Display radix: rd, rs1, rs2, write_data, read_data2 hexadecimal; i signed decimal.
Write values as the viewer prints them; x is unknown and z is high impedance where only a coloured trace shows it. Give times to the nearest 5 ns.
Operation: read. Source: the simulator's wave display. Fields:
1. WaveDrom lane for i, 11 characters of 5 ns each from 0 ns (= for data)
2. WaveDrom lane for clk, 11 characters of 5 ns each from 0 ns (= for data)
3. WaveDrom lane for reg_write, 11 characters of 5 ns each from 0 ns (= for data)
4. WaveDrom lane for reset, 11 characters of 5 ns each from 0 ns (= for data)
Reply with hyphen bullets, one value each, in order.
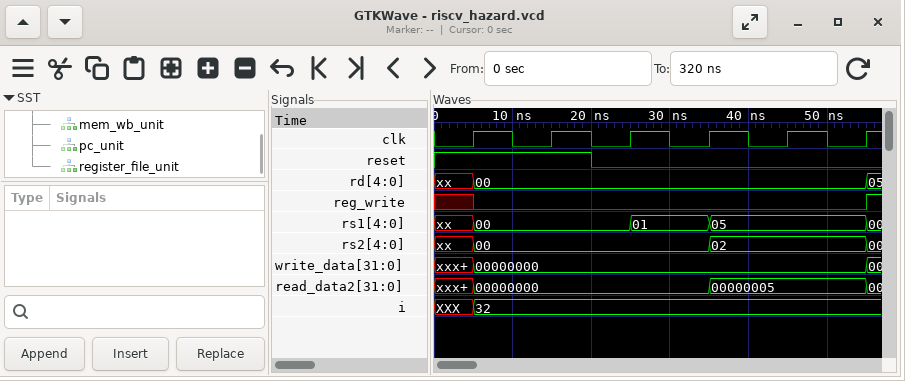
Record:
- {name: 'i', wave: 'x=.........', data: '32'}
- {name: 'clk', wave: '01010101010'}
- {name: 'reg_write', wave: 'x0.........'}
- {name: 'reset', wave: '1...0......'}
